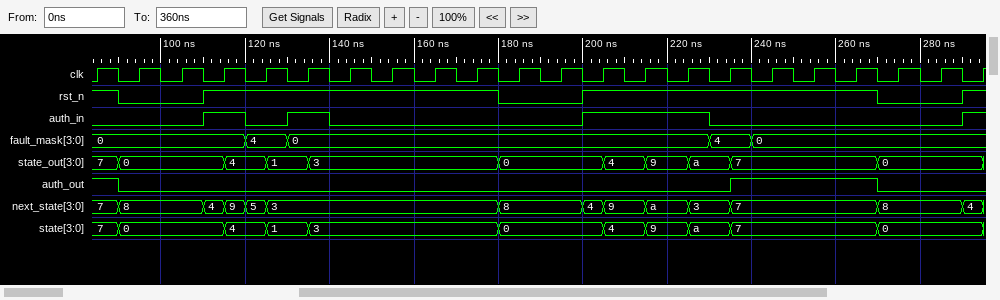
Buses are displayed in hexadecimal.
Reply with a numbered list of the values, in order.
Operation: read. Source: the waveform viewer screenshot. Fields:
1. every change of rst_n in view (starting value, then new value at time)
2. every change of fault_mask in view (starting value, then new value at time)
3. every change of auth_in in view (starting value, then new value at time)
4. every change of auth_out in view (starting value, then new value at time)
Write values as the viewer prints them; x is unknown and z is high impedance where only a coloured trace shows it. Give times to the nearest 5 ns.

1. 1, 0 at 90 ns, 1 at 110 ns, 0 at 180 ns, 1 at 200 ns, 0 at 270 ns, 1 at 290 ns
2. 0, 4 at 120 ns, 0 at 130 ns, 4 at 230 ns, 0 at 240 ns
3. 0, 1 at 110 ns, 0 at 120 ns, 1 at 130 ns, 0 at 140 ns, 1 at 200 ns, 0 at 230 ns, 1 at 290 ns
4. 1, 0 at 90 ns, 1 at 235 ns, 0 at 270 ns
